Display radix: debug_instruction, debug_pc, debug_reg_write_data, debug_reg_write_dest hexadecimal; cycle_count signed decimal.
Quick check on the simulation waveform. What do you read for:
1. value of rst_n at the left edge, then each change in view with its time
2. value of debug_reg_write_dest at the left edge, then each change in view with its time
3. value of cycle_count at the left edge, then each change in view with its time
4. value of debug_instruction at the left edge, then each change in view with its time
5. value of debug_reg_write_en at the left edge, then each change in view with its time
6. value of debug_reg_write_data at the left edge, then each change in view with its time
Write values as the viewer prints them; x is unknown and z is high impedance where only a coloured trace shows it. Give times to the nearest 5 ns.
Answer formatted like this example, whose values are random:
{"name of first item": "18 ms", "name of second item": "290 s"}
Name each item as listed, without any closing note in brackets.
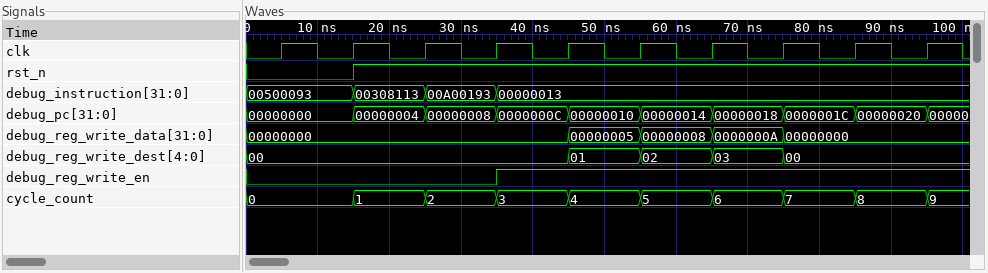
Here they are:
{"value of rst_n at the left edge, then each change in view with its time": "0, 1 at 15 ns", "value of debug_reg_write_dest at the left edge, then each change in view with its time": "00, 01 at 45 ns, 02 at 55 ns, 03 at 65 ns, 00 at 75 ns", "value of cycle_count at the left edge, then each change in view with its time": "0, 1 at 15 ns, 2 at 25 ns, 3 at 35 ns, 4 at 45 ns, 5 at 55 ns, 6 at 65 ns, 7 at 75 ns, 8 at 85 ns, 9 at 95 ns", "value of debug_instruction at the left edge, then each change in view with its time": "00500093, 00308113 at 15 ns, 00A00193 at 25 ns, 00000013 at 35 ns", "value of debug_reg_write_en at the left edge, then each change in view with its time": "0, 1 at 35 ns", "value of debug_reg_write_data at the left edge, then each change in view with its time": "00000000, 00000005 at 45 ns, 00000008 at 55 ns, 0000000A at 65 ns, 00000000 at 75 ns"}
